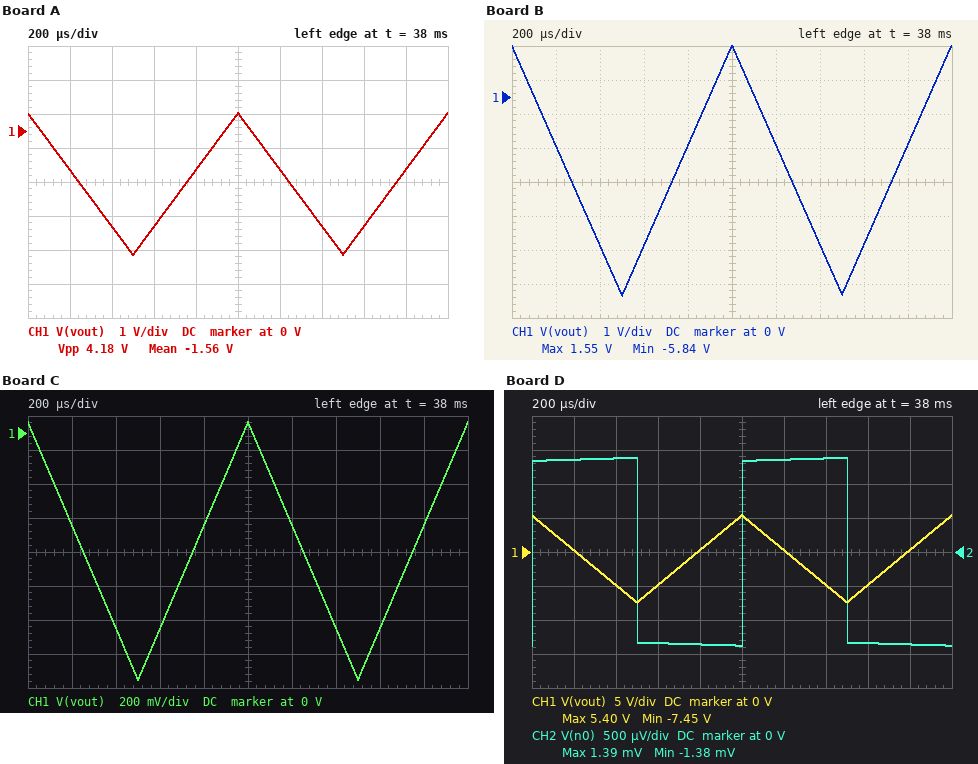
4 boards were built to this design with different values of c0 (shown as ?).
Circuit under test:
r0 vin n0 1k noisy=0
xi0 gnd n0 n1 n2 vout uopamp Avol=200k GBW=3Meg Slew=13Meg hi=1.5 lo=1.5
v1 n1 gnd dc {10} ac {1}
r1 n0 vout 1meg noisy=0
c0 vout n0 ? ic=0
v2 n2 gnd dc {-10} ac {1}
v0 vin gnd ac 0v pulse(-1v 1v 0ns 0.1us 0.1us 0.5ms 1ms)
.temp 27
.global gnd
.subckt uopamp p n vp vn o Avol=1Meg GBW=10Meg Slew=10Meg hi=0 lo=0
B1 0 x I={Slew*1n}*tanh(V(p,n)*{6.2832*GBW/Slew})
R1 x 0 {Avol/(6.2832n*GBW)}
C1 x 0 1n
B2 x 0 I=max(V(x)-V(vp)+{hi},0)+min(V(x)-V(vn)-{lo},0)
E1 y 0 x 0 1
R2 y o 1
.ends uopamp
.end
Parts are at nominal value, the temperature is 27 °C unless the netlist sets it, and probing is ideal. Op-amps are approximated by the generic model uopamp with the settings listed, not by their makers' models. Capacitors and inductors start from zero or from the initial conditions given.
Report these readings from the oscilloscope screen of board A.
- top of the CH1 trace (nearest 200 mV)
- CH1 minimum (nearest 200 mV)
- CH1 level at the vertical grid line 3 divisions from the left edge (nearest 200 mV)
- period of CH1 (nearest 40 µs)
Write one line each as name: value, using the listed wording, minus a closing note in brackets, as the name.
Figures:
top of the CH1 trace: 600 mV
CH1 minimum: -3.6 V
CH1 level at the vertical grid line 3 divisions from the left edge: -2.8 V
period of CH1: 1.00 ms
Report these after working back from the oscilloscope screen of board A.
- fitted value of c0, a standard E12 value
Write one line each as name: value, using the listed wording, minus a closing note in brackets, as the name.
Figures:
fitted value of c0, a standard E12 value: 120 nF
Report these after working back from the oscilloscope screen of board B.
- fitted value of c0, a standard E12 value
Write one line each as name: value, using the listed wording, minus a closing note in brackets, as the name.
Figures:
fitted value of c0, a standard E12 value: 68 nF
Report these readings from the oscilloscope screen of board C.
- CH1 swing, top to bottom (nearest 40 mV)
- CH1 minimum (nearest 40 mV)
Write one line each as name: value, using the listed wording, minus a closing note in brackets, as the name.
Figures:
CH1 swing, top to bottom: 1.52 V
CH1 minimum: -1.44 V
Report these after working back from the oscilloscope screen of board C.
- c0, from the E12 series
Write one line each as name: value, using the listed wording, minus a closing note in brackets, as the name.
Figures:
c0, from the E12 series: 330 nF
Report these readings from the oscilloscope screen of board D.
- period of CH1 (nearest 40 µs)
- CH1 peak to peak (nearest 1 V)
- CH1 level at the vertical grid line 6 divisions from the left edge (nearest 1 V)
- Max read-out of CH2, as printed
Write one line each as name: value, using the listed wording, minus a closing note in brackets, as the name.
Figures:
period of CH1: 1.00 ms
CH1 peak to peak: 13 V
CH1 level at the vertical grid line 6 divisions from the left edge: 0 V
Max read-out of CH2, as printed: 1.39 mV
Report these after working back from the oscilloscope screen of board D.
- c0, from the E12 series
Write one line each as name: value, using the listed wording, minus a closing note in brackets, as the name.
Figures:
c0, from the E12 series: 39 nF
